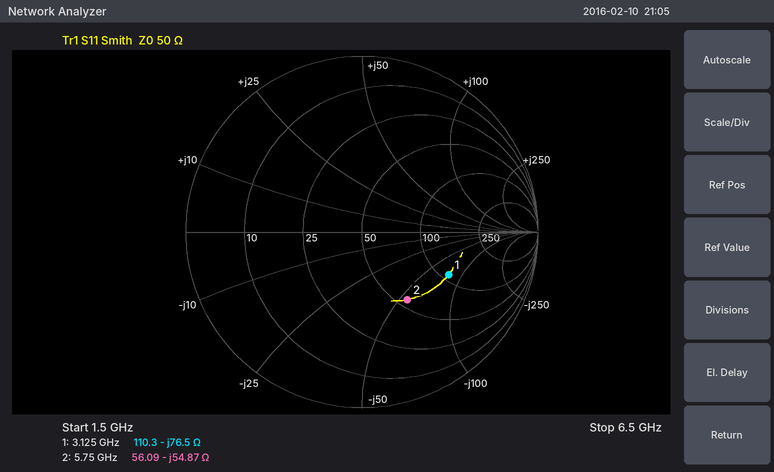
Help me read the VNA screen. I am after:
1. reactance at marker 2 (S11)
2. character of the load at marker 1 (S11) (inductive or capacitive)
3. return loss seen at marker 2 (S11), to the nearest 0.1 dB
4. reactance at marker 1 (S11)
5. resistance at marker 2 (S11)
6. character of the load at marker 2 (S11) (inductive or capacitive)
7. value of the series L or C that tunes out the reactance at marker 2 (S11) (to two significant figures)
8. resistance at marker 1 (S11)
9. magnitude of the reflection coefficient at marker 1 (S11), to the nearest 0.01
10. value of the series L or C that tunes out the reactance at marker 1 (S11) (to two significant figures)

-54.87 Ω
capacitive
6.7 dB
-76.5 Ω
56.09 Ω
capacitive
1.5 nH
110.3 Ω
0.55
3.9 nH
